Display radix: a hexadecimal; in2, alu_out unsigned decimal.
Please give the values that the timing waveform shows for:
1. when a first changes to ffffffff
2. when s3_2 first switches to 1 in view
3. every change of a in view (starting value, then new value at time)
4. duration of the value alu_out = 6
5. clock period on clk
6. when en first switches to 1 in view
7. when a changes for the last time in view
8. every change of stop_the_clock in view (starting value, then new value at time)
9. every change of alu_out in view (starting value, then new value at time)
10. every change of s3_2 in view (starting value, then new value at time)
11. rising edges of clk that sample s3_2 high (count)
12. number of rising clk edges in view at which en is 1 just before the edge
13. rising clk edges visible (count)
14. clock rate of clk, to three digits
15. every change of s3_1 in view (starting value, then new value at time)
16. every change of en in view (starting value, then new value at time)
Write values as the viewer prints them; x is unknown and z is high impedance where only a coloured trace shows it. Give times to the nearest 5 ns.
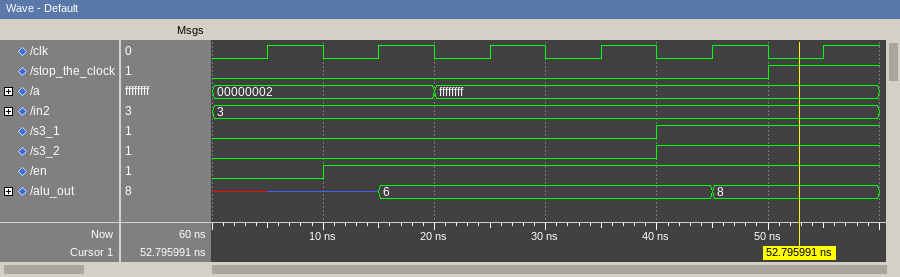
20 ns
40 ns
00000002, ffffffff at 20 ns
30 ns
10 ns
10 ns
20 ns
0, 1 at 50 ns
x, z at 5 ns, 6 at 15 ns, 8 at 45 ns
0, 1 at 40 ns
2
5
6
100 MHz
0, 1 at 40 ns
0, 1 at 10 ns
